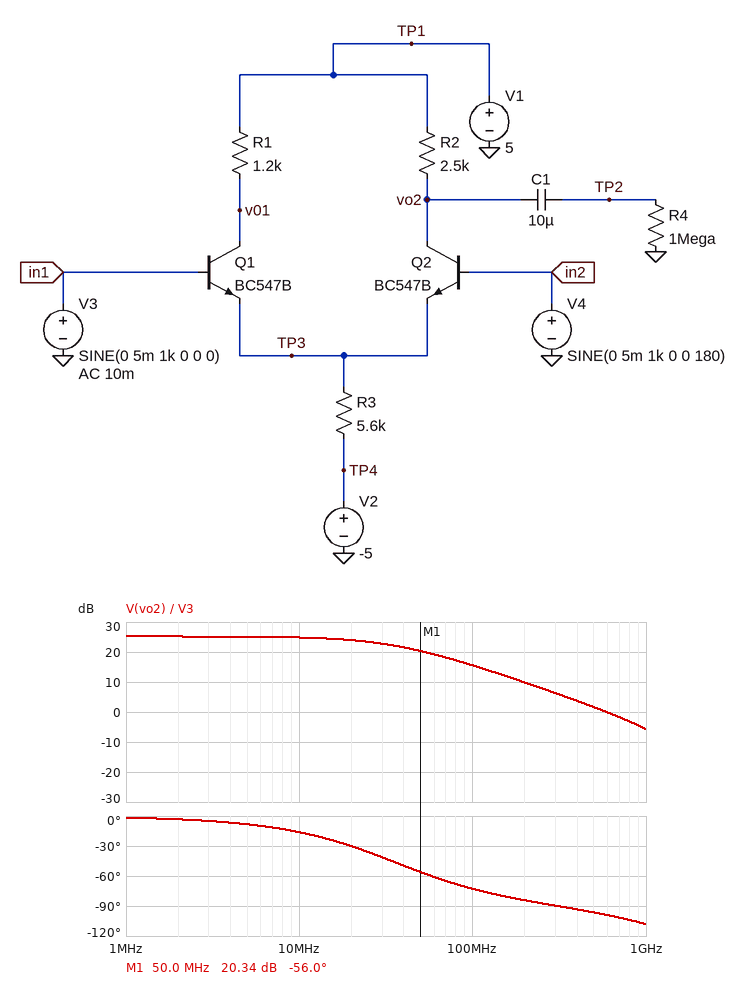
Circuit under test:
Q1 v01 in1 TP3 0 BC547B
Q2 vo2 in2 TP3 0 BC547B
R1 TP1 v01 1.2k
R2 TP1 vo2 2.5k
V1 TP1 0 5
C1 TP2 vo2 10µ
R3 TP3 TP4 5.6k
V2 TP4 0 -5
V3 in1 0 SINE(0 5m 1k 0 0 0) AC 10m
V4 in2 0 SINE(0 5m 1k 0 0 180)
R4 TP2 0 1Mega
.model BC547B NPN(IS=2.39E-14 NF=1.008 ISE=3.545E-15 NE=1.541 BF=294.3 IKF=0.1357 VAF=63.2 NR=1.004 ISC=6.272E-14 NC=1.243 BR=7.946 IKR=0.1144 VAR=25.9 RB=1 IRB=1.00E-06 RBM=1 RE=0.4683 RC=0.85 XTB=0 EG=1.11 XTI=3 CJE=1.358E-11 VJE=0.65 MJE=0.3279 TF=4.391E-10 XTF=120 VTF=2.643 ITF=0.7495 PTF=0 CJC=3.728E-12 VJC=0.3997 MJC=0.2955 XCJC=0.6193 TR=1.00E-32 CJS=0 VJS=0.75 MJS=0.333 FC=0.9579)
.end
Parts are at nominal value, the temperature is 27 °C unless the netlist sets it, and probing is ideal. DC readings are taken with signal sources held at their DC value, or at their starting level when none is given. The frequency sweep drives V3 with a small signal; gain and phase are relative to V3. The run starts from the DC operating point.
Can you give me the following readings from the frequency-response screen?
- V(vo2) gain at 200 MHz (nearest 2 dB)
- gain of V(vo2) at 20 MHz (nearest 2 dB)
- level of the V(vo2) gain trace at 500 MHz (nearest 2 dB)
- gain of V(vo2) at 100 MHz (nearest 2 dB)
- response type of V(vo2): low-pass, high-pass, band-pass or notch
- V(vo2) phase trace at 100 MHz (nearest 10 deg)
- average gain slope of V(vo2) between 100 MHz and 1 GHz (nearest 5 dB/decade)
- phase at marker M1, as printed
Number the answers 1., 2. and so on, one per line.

1. 10 dB
2. 24 dB
3. 2 dB
4. 16 dB
5. low-pass
6. -70 deg
7. -20 dB/decade
8. -56.0 deg
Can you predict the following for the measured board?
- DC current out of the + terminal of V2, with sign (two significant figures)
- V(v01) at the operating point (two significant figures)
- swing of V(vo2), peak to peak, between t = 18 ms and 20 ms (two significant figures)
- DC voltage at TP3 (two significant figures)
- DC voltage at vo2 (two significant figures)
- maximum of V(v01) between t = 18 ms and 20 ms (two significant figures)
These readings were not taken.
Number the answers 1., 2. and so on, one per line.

1. -780 µA
2. 4.5 V
3. 360 mV
4. -610 mV
5. 4.0 V
6. 4.6 V
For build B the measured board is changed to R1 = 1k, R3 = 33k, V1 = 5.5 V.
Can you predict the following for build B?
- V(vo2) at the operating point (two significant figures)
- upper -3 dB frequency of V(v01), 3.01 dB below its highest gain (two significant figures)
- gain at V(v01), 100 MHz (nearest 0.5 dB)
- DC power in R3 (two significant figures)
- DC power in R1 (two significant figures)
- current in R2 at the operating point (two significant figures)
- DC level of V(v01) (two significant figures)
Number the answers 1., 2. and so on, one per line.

1. 5.3 V
2. 4.0 GHz
3. 1.0 dB
4. 600 µW
5. 4.5 µW
6. 67 µA
7. 5.4 V
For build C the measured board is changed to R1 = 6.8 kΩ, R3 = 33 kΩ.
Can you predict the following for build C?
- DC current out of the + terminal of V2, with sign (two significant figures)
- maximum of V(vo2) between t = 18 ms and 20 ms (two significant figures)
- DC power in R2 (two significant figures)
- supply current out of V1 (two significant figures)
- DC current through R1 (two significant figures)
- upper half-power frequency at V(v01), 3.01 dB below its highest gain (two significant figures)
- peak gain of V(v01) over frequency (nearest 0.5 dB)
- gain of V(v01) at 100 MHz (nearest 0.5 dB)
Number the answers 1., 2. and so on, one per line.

1. -130 µA
2. 4.9 V
3. 11 µW
4. 130 µA
5. 67 µA
6. 13 MHz
7. 19.0 dB
8. 3.5 dB
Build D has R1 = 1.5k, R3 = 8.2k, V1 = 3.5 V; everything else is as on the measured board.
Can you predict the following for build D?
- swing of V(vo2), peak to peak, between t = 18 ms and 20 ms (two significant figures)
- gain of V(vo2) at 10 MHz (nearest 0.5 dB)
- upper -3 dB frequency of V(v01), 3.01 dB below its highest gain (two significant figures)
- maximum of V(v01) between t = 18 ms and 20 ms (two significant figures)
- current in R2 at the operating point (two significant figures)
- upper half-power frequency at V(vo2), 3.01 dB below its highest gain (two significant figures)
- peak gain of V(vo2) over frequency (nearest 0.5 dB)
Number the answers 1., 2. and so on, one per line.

1. 250 mV
2. 21.5 dB
3. 55 MHz
4. 3.2 V
5. 270 µA
6. 32 MHz
7. 22.0 dB
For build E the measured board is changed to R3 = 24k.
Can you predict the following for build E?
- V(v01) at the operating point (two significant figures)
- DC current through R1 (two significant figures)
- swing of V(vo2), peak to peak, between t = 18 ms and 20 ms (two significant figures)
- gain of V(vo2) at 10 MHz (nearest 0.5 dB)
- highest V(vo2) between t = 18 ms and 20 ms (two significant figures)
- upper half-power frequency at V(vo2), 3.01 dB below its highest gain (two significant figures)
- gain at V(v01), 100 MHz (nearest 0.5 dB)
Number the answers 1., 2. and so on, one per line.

1. 4.9 V
2. 92 µA
3. 86 mV
4. 12.5 dB
5. 4.8 V
6. 37 MHz
7. 3.5 dB
